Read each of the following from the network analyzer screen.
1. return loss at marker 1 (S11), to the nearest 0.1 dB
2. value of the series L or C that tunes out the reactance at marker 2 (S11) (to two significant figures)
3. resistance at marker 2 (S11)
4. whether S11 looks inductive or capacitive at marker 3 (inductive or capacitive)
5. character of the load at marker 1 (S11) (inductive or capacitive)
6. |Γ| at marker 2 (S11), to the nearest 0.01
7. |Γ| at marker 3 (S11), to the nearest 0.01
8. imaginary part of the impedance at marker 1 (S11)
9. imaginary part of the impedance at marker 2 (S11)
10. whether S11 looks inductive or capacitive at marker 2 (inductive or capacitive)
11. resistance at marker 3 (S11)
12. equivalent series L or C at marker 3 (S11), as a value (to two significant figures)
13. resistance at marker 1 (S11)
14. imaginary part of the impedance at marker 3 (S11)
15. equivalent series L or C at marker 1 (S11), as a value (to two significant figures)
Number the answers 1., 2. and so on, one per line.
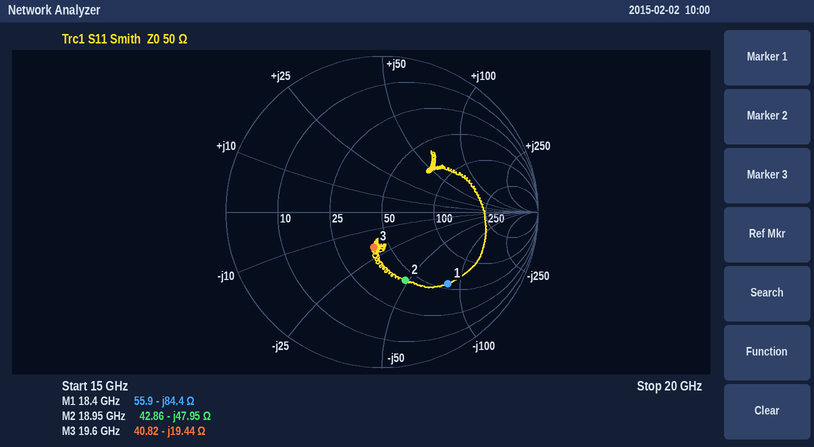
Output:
1. 4.1 dB
2. 400 pH
3. 42.86 Ω
4. capacitive
5. capacitive
6. 0.46
7. 0.23
8. -84.4 Ω
9. -47.95 Ω
10. capacitive
11. 40.82 Ω
12. 420 fF
13. 55.9 Ω
14. -19.44 Ω
15. 100 fF
